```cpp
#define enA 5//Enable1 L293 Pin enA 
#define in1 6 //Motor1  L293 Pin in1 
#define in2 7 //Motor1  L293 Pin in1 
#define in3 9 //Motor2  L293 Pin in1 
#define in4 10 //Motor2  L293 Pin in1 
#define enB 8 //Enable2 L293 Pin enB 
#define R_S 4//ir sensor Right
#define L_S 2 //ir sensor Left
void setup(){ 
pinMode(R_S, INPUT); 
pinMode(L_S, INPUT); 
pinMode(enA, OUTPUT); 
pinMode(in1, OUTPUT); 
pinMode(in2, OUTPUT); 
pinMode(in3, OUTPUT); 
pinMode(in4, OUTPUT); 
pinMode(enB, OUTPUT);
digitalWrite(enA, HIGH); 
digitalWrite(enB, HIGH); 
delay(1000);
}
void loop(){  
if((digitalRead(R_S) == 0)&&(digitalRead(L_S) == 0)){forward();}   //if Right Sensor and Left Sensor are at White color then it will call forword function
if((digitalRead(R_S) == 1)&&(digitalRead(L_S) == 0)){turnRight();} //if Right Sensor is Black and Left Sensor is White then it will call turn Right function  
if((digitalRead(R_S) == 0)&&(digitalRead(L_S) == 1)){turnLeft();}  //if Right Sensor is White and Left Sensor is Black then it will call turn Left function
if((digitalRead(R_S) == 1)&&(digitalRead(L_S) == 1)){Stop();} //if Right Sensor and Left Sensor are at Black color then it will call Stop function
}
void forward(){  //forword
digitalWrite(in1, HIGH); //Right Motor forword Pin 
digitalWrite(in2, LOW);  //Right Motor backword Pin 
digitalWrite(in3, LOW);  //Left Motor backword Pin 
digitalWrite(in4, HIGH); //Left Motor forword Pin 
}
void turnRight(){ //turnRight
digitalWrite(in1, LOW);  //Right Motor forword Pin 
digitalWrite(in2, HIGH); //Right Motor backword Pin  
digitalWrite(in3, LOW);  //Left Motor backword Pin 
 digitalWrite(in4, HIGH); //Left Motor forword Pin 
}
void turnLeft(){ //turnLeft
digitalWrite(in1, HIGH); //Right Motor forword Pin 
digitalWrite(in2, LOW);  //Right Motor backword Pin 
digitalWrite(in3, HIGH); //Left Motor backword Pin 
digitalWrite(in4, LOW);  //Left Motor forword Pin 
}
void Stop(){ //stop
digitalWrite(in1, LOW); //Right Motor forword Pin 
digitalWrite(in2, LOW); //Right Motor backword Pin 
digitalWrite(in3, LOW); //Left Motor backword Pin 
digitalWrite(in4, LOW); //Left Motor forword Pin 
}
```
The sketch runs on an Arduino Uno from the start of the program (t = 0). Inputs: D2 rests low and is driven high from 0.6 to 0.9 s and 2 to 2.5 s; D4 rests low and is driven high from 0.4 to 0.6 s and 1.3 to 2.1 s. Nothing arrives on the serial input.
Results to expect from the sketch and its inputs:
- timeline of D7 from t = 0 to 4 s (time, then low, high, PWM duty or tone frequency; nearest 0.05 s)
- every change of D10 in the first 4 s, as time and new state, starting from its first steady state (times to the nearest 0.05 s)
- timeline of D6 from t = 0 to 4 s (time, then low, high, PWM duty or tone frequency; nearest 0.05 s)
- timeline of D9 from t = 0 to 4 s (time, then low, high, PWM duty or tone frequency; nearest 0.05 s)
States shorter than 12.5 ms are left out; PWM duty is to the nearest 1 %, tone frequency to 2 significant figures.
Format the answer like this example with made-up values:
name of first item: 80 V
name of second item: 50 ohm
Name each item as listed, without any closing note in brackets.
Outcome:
timeline of D7 from t = 0 to 4 s: 0 s low; 1.3 s high; 2 s low
every change of D10 in the first 4 s, as time and new state, starting from its first steady state: 0 s low; 1 s high; 2 s low; 2.5 s high
timeline of D6 from t = 0 to 4 s: 0 s low; 1 s high; 1.3 s low; 2.1 s high
timeline of D9 from t = 0 to 4 s: 0 s low; 2.1 s high; 2.5 s low
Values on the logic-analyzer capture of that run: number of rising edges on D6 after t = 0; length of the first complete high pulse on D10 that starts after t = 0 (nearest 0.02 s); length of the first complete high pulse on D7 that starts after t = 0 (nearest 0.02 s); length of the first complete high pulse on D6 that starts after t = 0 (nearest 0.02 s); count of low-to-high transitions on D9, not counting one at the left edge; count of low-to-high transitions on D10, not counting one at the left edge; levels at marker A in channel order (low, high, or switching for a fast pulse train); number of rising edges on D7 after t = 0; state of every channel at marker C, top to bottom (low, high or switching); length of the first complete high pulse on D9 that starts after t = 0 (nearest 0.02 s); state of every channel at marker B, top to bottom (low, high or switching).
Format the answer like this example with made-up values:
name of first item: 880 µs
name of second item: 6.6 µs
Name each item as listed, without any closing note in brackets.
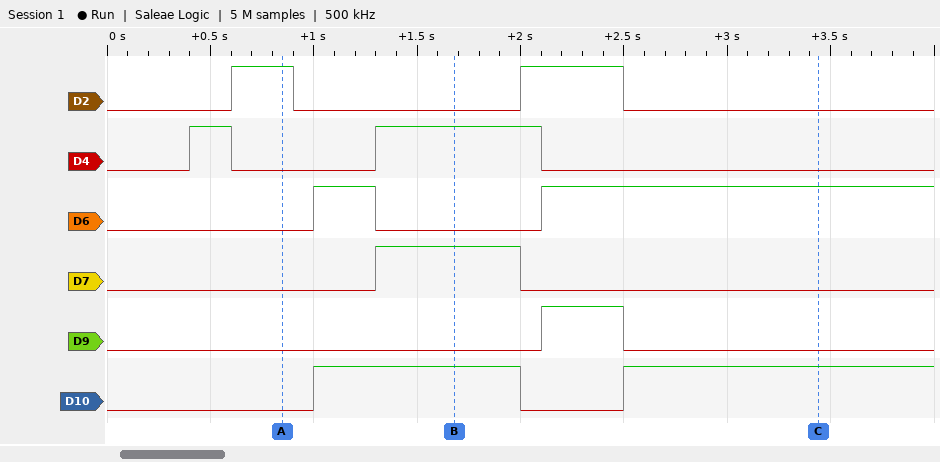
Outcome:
number of rising edges on D6 after t = 0: 2
length of the first complete high pulse on D10 that starts after t = 0: 1.00 s
length of the first complete high pulse on D7 that starts after t = 0: 0.70 s
length of the first complete high pulse on D6 that starts after t = 0: 0.30 s
count of low-to-high transitions on D9, not counting one at the left edge: 1
count of low-to-high transitions on D10, not counting one at the left edge: 2
levels at marker A in channel order: D2 high, D4 low, D6 low, D7 low, D9 low, D10 low
number of rising edges on D7 after t = 0: 1
state of every channel at marker C, top to bottom: D2 low, D4 low, D6 high, D7 low, D9 low, D10 high
length of the first complete high pulse on D9 that starts after t = 0: 0.40 s
state of every channel at marker B, top to bottom: D2 low, D4 high, D6 low, D7 high, D9 low, D10 high
